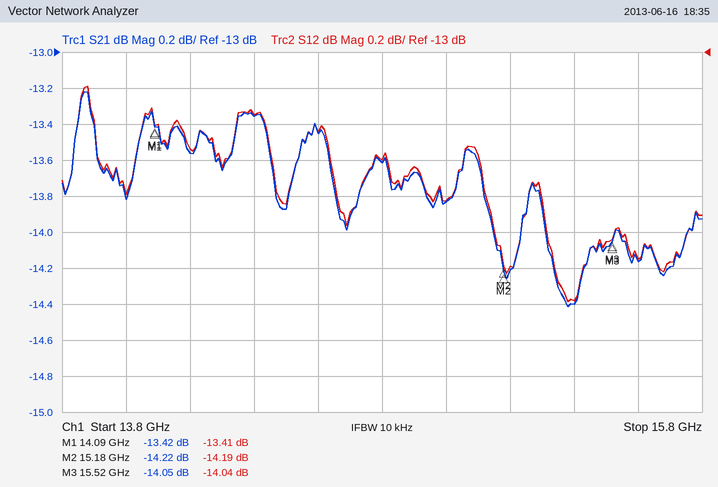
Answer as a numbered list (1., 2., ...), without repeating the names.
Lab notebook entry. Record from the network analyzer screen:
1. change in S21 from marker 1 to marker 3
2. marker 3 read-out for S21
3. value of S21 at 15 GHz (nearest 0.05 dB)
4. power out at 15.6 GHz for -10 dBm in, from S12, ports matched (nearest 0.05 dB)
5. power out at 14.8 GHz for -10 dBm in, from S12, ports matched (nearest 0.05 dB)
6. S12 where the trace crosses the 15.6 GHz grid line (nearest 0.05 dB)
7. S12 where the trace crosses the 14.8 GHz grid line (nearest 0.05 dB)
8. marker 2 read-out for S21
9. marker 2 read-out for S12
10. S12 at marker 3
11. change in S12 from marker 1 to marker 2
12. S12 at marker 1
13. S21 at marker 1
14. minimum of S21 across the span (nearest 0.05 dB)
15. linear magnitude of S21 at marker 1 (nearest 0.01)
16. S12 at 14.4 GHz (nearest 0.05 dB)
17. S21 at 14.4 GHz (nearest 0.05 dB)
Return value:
1. -0.63 dB
2. -14.05 dB
3. -13.85 dB
4. -24.15 dBm
5. -23.60 dBm
6. -14.15 dB
7. -13.60 dB
8. -14.22 dB
9. -14.19 dB
10. -14.04 dB
11. -0.78 dB
12. -13.41 dB
13. -13.42 dB
14. -14.40 dB
15. 0.21
16. -13.35 dB
17. -13.35 dB
